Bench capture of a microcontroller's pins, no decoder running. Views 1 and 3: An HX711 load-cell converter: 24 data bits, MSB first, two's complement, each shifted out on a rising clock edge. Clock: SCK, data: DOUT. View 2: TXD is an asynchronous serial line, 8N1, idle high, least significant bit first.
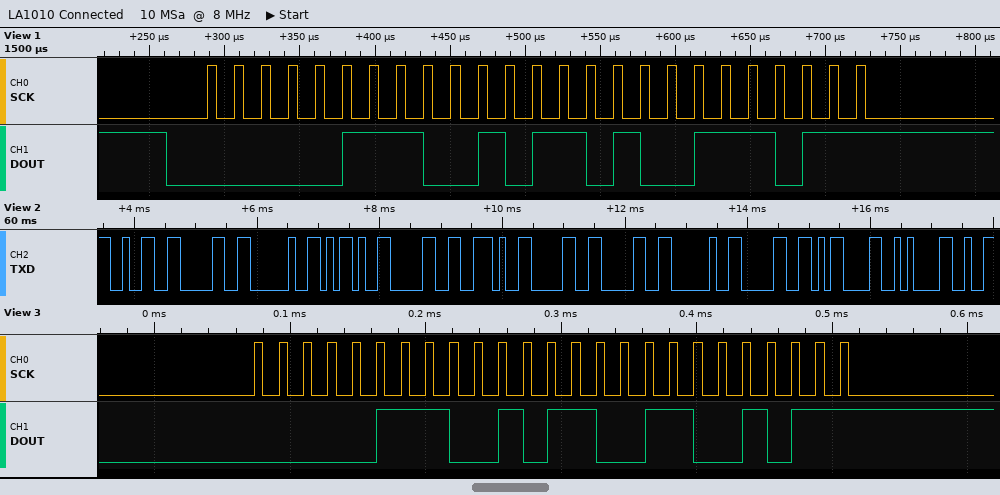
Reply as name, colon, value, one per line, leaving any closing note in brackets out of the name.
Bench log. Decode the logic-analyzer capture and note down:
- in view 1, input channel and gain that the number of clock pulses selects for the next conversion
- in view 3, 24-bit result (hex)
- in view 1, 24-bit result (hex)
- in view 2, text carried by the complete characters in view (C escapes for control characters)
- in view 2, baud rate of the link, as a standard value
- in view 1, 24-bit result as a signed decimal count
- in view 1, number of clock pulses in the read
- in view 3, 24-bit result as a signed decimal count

in view 1, input channel and gain that the number of clock pulses selects for the next conversion: channel A, gain 128
in view 3, 24-bit result: 0x072CCB
in view 1, 24-bit result: 0x072D3B
in view 2, text carried by the complete characters in view: "20 -0.00 0\r\n"
in view 2, baud rate of the link, as a standard value: 9600 baud
in view 1, 24-bit result as a signed decimal count: 470331
in view 1, number of clock pulses in the read: 25
in view 3, 24-bit result as a signed decimal count: 470219
